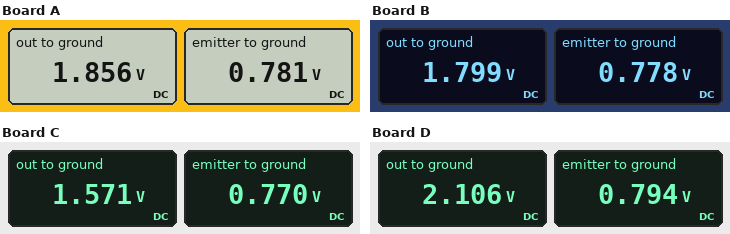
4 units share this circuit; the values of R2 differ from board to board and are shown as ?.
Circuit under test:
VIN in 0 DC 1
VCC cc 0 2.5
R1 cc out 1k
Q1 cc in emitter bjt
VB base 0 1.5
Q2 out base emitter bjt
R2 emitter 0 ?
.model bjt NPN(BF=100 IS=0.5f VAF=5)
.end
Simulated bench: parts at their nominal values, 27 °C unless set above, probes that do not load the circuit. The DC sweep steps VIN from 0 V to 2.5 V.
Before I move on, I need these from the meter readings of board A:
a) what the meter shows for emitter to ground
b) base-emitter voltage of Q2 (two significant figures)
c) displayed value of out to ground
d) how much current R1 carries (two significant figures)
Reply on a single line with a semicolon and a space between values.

0.781 V; 720 mV; 1.856 V; 640 µA
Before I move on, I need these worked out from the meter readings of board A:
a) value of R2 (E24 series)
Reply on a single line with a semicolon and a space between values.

1.2 kΩ
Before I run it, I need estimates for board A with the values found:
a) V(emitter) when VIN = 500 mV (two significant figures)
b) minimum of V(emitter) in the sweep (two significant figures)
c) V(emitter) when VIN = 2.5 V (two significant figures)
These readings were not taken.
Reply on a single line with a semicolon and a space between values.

780 mV; 780 mV; 1.8 V
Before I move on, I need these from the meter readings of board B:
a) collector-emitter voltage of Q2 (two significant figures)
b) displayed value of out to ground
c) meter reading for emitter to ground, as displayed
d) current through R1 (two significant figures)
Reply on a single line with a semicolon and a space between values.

1.0 V; 1.799 V; 0.778 V; 700 µA
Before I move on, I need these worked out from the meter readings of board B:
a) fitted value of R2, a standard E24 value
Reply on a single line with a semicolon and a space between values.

1.1 kΩ
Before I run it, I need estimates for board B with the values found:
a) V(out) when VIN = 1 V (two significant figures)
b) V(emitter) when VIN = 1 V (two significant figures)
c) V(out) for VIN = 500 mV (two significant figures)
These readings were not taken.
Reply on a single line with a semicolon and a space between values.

1.8 V; 780 mV; 1.8 V
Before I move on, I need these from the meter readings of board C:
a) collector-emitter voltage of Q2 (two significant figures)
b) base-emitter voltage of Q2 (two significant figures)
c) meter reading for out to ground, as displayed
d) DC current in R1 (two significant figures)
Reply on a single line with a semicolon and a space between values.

800 mV; 730 mV; 1.571 V; 930 µA
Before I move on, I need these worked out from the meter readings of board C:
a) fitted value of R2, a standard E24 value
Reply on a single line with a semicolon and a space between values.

820 Ω
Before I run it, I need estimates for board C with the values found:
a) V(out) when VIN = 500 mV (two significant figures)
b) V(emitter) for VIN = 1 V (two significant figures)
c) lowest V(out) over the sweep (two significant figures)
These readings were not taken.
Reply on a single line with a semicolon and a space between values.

1.6 V; 770 mV; 1.6 V
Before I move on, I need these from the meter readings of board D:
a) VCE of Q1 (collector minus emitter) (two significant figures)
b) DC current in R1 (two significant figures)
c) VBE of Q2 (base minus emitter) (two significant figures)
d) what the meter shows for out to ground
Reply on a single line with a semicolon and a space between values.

1.7 V; 390 µA; 710 mV; 2.106 V
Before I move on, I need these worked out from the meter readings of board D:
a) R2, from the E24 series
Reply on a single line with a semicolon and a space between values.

2 kΩ
